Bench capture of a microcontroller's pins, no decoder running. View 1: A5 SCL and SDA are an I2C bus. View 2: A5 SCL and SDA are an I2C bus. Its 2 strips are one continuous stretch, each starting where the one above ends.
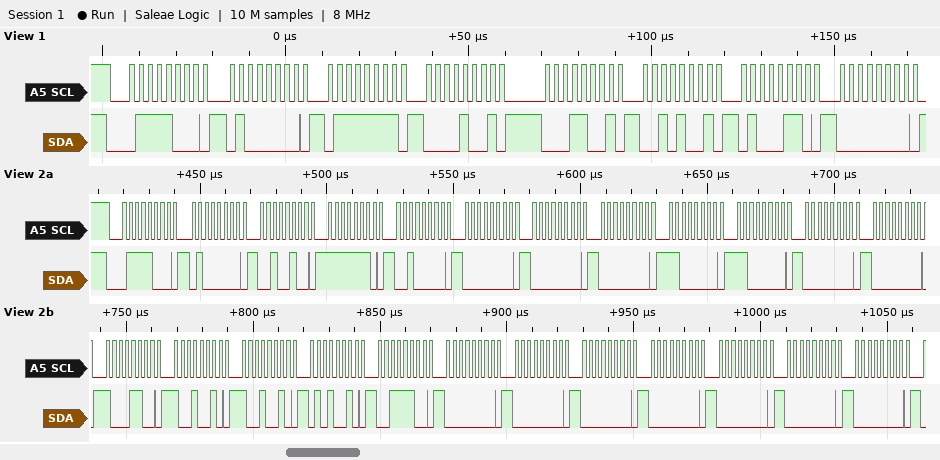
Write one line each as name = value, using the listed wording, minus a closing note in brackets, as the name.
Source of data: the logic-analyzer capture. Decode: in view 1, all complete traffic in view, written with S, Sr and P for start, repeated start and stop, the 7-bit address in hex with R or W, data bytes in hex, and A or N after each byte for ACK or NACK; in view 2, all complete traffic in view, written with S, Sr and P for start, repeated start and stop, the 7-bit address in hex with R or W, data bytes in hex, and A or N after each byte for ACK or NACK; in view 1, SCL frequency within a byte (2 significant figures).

in view 1, all complete traffic in view, written with S, Sr and P for start, repeated start and stop, the 7-bit address in hex with R or W, data bytes in hex, and A or N after each byte for ACK or NACK = S 3CW A 40 A 7F A 09 A 19 A 29 A 46 A 00 A
in view 2, all complete traffic in view, written with S, Sr and P for start, repeated start and stop, the 7-bit address in hex with R or W, data bytes in hex, and A or N after each byte for ACK or NACK = S 3CW A 40 A 24 A FE A 20 A 00 A 00 A 00 A C0 A C0 A 00 A 00 A 8C A 92 A 92 A 52 A 3C A 00 A 00 A 00 A 00 A 00 A 00 A 00 A
in view 1, SCL frequency within a byte = 400 kHz
